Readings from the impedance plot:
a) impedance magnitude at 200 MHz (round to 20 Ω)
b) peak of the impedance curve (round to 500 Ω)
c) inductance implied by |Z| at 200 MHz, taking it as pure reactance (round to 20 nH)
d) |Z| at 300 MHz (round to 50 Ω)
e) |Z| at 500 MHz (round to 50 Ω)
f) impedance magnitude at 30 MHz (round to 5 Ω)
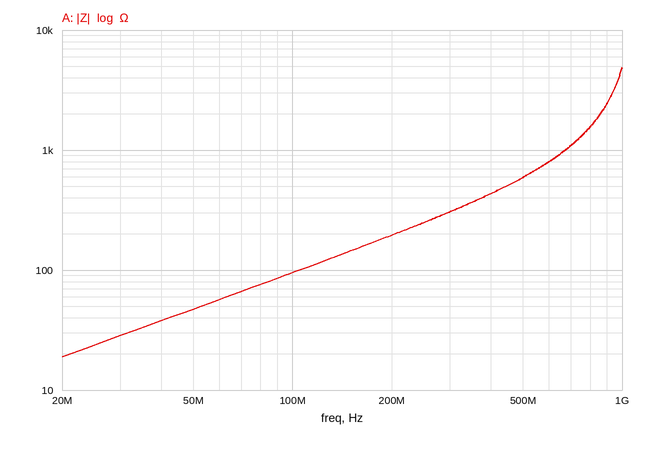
200 Ω
5.0 kΩ
160 nH
300 Ω
600 Ω
30 Ω
